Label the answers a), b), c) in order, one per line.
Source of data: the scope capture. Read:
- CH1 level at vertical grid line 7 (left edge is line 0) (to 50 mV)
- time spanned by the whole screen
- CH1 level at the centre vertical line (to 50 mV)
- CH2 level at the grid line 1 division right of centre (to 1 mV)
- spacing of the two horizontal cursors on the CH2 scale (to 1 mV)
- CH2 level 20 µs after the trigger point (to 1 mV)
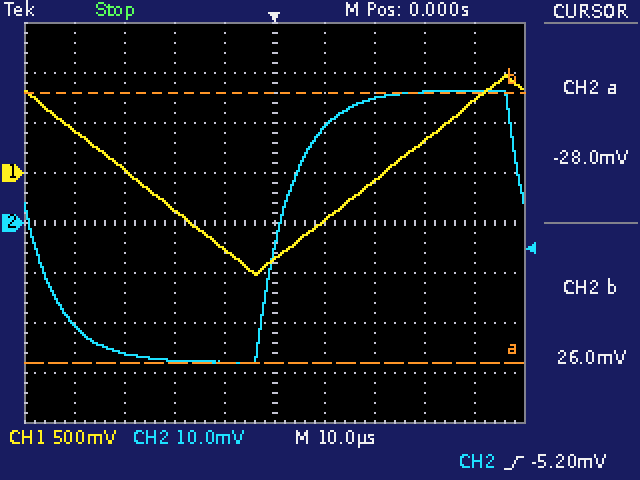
a) -100 mV
b) 100 µs
c) -850 mV
d) 19 mV
e) 54 mV
f) 25 mV
